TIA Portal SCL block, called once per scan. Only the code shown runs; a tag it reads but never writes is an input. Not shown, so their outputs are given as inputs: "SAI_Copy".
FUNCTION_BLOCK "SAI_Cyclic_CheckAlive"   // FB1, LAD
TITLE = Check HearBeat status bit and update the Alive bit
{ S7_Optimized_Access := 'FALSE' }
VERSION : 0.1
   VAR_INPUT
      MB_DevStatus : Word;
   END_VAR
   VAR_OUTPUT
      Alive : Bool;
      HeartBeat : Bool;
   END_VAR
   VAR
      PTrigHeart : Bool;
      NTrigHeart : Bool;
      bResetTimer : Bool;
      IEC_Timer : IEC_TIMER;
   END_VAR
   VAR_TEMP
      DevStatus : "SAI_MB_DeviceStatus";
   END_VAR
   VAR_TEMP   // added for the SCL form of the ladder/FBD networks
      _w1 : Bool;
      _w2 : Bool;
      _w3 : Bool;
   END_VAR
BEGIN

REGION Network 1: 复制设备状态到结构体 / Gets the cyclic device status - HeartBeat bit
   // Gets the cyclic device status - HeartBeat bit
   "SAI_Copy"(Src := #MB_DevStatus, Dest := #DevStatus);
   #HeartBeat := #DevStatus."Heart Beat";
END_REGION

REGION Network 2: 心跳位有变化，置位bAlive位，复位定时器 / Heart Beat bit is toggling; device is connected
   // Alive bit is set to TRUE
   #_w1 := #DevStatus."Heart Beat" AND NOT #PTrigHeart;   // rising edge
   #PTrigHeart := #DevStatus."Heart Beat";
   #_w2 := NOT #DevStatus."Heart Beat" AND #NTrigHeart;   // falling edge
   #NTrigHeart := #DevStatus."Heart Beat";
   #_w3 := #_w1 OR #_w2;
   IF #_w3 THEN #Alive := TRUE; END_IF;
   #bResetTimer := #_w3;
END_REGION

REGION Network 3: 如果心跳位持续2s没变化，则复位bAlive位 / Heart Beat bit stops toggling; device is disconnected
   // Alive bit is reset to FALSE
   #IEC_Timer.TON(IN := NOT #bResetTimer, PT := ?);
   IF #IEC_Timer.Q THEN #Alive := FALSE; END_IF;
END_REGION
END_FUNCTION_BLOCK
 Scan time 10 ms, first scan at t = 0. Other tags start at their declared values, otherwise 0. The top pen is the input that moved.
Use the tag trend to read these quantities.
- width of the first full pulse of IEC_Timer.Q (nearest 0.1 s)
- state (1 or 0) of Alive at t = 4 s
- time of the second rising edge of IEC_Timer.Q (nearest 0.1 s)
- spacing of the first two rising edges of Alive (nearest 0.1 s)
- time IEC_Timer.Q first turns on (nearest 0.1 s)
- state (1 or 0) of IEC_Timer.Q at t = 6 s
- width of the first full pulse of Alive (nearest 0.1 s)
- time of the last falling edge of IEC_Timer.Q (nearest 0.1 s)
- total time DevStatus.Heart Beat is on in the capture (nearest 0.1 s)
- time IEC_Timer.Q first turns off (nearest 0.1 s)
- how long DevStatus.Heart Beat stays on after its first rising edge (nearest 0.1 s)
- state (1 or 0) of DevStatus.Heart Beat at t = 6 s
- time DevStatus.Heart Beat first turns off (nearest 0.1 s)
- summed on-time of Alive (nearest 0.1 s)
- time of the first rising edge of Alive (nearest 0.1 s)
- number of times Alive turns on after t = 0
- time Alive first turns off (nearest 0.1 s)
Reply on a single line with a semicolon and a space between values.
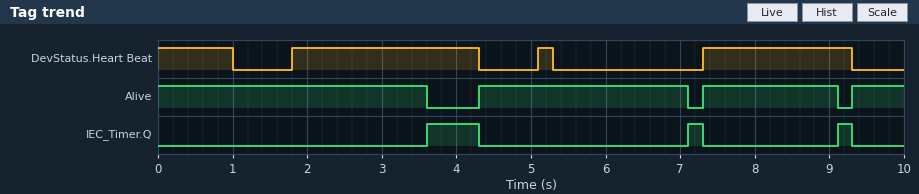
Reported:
0.7 s; 0; 7.1 s; 3.0 s; 3.6 s; 0; 2.8 s; 9.3 s; 5.7 s; 4.3 s; 2.5 s; 0; 1.0 s; 8.9 s; 4.3 s; 3; 3.6 s
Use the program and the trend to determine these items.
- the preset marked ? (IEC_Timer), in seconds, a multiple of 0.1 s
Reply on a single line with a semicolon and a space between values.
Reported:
1.8 s
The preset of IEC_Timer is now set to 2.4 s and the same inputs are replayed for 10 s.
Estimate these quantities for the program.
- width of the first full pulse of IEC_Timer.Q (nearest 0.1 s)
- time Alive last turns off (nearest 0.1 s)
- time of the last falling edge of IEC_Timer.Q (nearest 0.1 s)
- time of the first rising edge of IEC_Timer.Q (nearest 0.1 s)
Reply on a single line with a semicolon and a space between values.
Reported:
0.1 s; 4.2 s; 4.3 s; 4.2 s
